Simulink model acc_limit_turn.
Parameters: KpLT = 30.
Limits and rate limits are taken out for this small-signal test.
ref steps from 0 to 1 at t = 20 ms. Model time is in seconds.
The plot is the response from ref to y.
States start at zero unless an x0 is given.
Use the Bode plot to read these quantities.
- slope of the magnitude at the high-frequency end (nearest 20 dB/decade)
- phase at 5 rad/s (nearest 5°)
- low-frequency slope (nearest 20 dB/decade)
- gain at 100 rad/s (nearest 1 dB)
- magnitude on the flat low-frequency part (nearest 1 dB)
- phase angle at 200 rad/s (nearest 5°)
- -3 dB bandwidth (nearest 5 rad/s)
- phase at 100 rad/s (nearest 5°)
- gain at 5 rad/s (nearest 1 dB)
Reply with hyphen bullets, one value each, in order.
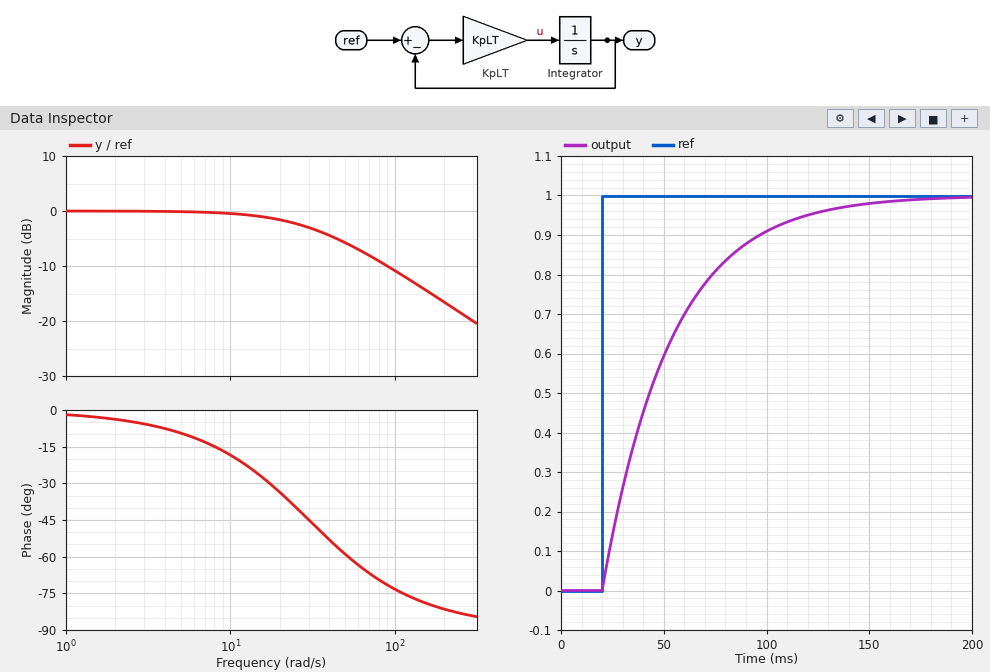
- -20 dB/decade
- -10°
- 0 dB/decade
- -11 dB
- 0 dB
- -80°
- 30 rad/s
- -75°
- 0 dB
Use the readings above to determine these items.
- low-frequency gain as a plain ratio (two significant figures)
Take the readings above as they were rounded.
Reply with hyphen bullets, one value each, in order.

- 1.0
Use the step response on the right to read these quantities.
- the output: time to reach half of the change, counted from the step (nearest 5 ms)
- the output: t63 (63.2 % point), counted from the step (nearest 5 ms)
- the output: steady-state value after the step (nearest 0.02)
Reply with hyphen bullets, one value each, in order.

- 25 ms
- 35 ms
- 1.00
